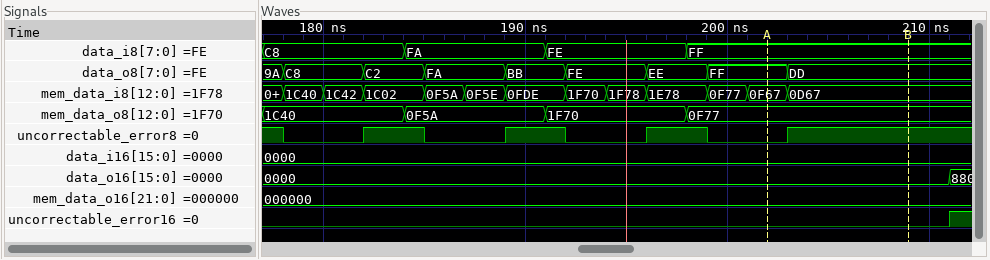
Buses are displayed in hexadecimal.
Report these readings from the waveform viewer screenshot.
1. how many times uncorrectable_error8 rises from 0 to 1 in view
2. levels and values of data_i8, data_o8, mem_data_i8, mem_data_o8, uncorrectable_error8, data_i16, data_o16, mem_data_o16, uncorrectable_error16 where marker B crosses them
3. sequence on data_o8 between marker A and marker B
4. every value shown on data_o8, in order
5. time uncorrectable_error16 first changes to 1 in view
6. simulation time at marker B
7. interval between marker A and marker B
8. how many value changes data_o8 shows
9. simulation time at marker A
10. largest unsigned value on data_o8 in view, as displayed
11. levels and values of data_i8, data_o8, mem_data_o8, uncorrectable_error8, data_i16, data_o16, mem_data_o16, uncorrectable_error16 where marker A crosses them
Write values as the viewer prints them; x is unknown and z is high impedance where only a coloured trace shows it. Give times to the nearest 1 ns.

4
data_i8=FF, data_o8=DD, mem_data_i8=0D67, mem_data_o8=0F77, uncorrectable_error8=1, data_i16=0000, data_o16=0000, mem_data_o16=000000, uncorrectable_error16=0
FF, DD
9A, C8, C2, FA, BB, FE, EE, FF, DD
211 ns
209 ns
7 ns
8
202 ns
FF
data_i8=FF, data_o8=FF, mem_data_o8=0F77, uncorrectable_error8=0, data_i16=0000, data_o16=0000, mem_data_o16=000000, uncorrectable_error16=0
